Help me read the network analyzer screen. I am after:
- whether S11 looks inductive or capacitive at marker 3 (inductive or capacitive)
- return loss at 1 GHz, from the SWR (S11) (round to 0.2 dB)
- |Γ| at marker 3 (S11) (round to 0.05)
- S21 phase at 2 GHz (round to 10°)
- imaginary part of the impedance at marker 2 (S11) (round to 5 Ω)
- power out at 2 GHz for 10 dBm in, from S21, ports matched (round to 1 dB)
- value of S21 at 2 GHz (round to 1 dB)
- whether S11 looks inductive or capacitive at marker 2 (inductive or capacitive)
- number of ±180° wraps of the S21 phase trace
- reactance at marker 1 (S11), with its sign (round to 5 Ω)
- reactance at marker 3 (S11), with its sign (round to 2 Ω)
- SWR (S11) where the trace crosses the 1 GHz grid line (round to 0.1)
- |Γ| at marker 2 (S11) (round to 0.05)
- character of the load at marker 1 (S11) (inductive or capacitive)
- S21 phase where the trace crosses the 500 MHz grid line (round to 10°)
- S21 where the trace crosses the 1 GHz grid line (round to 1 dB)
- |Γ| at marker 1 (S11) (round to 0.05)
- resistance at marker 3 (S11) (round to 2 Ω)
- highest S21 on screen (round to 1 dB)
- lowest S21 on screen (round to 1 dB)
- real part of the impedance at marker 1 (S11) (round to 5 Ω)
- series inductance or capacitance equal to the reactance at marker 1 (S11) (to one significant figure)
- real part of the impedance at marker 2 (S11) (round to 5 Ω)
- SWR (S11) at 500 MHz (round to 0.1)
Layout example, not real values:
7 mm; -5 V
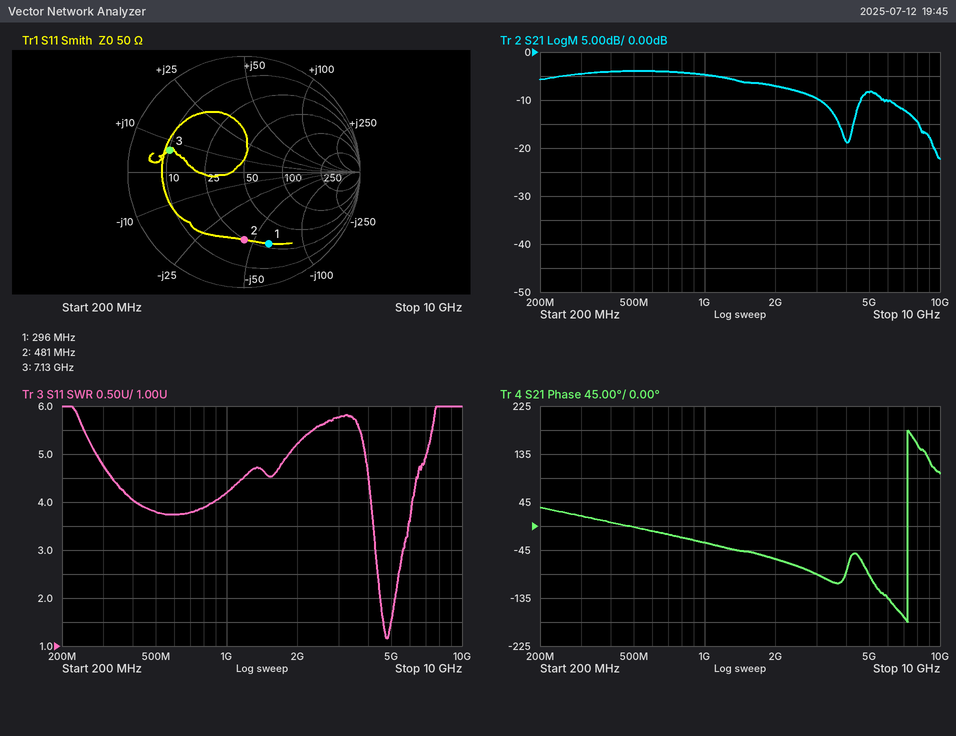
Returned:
inductive; 4.2 dB; 0.65; -60°; -45 Ω; 3 dBm; -7 dB; capacitive; 1; -60 Ω; +6 Ω; 4.2; 0.60; capacitive; 0°; -5 dB; 0.65; 10 Ω; -4 dB; -22 dB; 30 Ω; 9 pF; 25 Ω; 3.8
